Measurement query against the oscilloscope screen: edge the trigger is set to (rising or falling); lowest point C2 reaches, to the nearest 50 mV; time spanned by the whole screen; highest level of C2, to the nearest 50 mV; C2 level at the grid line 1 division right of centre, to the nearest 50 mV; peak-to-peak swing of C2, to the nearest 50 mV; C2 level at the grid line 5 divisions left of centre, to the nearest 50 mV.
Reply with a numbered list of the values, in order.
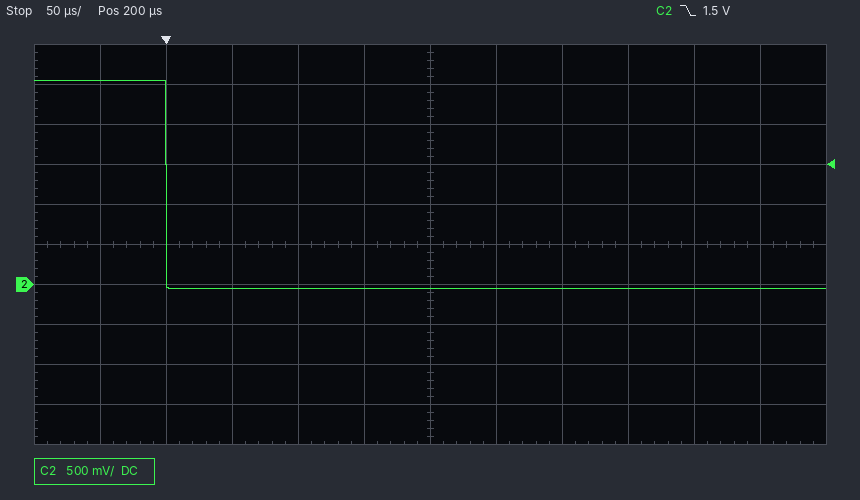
1. falling
2. -50 mV
3. 600 µs
4. 2.55 V
5. -50 mV
6. 2.60 V
7. 2.55 V
